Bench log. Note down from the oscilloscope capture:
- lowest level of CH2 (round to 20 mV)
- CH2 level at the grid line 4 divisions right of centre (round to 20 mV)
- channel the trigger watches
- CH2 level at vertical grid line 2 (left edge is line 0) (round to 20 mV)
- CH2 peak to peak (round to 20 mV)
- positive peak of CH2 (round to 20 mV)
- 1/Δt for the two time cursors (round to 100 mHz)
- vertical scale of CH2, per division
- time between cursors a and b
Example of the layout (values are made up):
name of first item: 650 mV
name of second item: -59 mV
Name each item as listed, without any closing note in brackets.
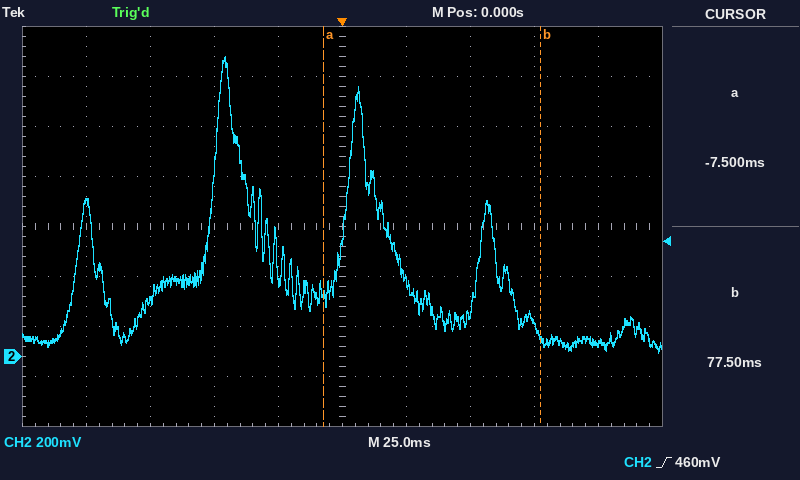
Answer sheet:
lowest level of CH2: 20 mV
CH2 level at the grid line 4 divisions right of centre: 60 mV
channel the trigger watches: CH2
CH2 level at vertical grid line 2 (left edge is line 0): 220 mV
CH2 peak to peak: 1.18 V
positive peak of CH2: 1.20 V
1/Δt for the two time cursors: 11.8 Hz
vertical scale of CH2, per division: 200 mV
time between cursors a and b: 85.0 ms
